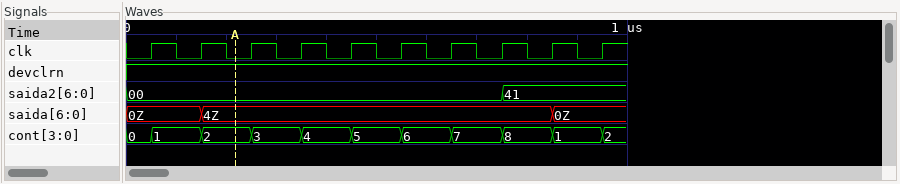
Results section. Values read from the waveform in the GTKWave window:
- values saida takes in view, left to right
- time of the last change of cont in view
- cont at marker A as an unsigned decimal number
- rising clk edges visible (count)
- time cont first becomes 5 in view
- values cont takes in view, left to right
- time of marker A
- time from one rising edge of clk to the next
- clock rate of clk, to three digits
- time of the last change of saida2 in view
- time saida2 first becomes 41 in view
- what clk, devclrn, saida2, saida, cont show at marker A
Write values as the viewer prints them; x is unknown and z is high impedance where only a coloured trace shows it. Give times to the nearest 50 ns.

0Z, 4Z, 0Z
950 ns
2
10
450 ns
0, 1, 2, 3, 4, 5, 6, 7, 8, 1, 2
200 ns
100 ns
10.0 MHz
750 ns
750 ns
clk=0, devclrn=1, saida2=00, saida=4Z, cont=2
